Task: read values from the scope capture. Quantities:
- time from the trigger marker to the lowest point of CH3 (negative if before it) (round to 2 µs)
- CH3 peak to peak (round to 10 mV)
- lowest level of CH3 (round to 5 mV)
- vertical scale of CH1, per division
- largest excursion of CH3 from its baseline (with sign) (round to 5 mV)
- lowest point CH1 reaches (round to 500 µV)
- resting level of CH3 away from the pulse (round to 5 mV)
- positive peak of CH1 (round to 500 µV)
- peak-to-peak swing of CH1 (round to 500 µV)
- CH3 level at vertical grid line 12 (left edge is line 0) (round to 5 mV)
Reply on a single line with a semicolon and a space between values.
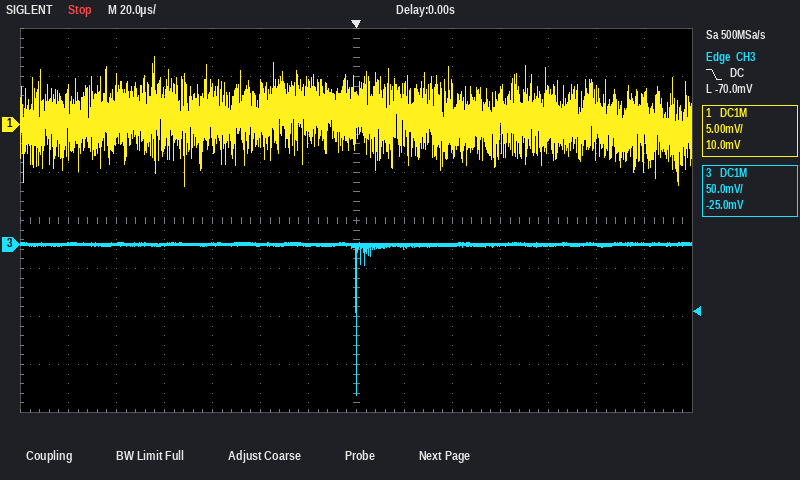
0 µs; 160 mV; -155 mV; 5 mV; -155 mV; -6.5 mV; 0 mV; 7.0 mV; 13.5 mV; 0 mV
